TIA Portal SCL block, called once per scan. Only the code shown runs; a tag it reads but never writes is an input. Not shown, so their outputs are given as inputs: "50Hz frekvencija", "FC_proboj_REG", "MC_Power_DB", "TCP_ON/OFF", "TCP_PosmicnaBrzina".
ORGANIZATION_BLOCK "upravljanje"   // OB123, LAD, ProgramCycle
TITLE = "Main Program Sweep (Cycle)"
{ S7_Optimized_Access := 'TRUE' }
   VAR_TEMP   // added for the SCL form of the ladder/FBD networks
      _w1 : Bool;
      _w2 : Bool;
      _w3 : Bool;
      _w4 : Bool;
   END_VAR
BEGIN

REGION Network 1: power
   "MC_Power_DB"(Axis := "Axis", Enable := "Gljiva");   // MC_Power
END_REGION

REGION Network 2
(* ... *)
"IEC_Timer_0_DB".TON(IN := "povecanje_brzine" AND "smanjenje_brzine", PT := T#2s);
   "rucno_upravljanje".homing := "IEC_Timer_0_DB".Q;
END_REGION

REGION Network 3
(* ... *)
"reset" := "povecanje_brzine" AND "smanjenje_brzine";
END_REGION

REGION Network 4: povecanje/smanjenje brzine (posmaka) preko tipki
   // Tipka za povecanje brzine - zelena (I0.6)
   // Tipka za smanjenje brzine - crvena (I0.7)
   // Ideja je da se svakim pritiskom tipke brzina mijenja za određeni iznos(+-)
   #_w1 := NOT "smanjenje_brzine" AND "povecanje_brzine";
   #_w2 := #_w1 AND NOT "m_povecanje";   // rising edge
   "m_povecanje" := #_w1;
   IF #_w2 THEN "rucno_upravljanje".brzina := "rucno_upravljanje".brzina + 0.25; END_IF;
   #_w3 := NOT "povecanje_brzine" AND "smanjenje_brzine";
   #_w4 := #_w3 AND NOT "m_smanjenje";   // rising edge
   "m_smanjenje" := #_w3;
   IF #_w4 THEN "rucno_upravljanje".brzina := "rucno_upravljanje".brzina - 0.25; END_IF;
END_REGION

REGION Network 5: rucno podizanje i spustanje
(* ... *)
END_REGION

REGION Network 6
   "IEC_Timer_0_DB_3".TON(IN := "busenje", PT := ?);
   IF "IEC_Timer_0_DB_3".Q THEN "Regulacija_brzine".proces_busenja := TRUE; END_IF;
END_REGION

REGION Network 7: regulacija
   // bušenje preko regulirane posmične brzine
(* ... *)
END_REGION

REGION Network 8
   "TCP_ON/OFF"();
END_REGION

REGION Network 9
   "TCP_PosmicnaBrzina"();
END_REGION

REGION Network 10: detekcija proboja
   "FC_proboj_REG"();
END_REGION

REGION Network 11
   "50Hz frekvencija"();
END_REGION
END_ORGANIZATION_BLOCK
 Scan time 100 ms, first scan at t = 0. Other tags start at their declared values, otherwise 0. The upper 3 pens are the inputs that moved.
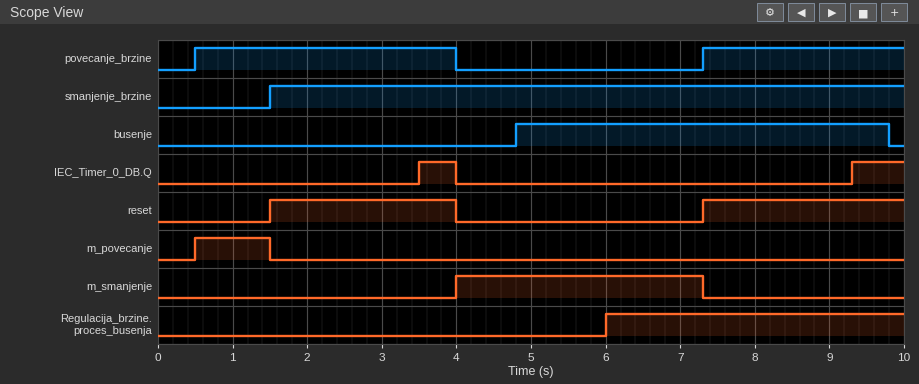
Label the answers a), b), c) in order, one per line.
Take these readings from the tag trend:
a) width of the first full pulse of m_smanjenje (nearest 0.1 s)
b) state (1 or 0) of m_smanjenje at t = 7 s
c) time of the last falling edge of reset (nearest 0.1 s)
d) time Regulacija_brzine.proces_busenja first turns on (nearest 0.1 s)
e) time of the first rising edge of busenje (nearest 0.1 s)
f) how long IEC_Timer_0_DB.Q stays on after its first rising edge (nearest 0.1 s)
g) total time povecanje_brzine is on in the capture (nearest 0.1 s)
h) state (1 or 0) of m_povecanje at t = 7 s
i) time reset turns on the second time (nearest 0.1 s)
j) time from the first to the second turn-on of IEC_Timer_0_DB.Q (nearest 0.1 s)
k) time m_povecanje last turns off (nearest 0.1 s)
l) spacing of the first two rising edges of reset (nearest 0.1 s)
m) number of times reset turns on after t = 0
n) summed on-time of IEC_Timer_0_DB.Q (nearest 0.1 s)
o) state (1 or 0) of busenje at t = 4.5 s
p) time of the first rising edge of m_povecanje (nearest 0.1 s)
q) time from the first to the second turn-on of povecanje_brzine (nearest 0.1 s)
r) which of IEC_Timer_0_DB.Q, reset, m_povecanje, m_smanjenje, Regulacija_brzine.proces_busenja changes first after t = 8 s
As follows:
a) 3.3 s
b) 1
c) 4.0 s
d) 6.0 s
e) 4.8 s
f) 0.5 s
g) 6.2 s
h) 0
i) 7.3 s
j) 5.8 s
k) 1.5 s
l) 5.8 s
m) 2
n) 1.2 s
o) 0
p) 0.5 s
q) 6.8 s
r) IEC_Timer_0_DB.Q
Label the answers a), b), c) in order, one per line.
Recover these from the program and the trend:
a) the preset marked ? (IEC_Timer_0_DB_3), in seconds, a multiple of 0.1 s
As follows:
a) 1.2 s
